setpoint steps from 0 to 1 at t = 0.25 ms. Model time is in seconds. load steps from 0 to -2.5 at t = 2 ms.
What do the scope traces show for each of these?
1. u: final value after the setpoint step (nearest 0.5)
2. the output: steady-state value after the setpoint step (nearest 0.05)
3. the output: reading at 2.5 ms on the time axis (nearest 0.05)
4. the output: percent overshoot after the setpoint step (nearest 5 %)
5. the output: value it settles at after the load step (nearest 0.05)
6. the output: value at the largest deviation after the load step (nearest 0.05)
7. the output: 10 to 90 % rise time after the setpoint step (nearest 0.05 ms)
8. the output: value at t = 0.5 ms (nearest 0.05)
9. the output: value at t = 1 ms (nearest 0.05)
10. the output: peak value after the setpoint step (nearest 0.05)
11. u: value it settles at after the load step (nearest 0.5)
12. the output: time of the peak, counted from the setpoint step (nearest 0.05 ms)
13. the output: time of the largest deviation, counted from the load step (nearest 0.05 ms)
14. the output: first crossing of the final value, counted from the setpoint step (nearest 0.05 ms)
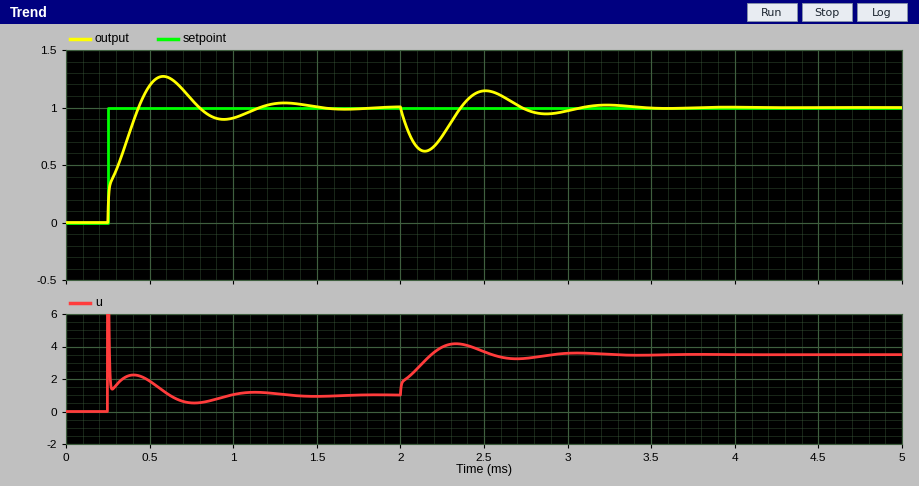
1.0
1.00
1.15
25 %
1.00
0.60
0.15 ms
1.20
0.90
1.25
3.5
0.35 ms
0.15 ms
0.20 ms
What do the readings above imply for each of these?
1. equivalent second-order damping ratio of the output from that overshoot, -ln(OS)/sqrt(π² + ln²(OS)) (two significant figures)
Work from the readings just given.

0.40
